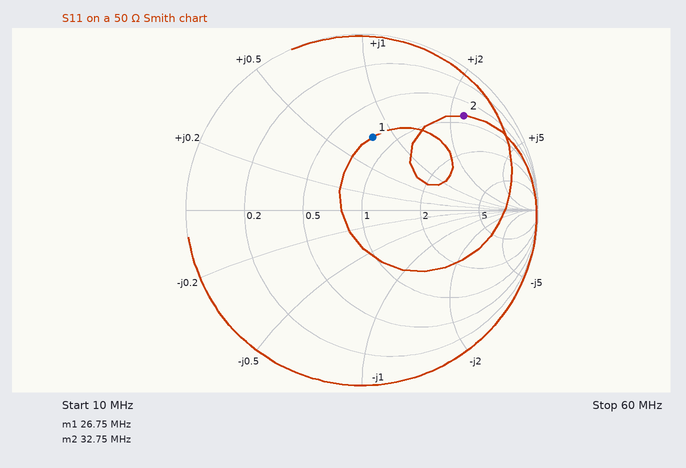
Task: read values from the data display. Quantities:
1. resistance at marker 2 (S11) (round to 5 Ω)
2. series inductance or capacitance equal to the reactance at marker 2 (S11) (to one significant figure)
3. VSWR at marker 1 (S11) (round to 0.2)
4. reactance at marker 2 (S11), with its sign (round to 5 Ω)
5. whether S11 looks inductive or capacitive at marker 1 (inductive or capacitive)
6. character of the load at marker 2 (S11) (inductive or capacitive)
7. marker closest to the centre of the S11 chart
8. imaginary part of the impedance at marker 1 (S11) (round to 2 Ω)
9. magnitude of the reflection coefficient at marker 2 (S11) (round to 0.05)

40 Ω
600 nH
2.4
+115 Ω
inductive
inductive
marker 1
+40 Ω
0.80
